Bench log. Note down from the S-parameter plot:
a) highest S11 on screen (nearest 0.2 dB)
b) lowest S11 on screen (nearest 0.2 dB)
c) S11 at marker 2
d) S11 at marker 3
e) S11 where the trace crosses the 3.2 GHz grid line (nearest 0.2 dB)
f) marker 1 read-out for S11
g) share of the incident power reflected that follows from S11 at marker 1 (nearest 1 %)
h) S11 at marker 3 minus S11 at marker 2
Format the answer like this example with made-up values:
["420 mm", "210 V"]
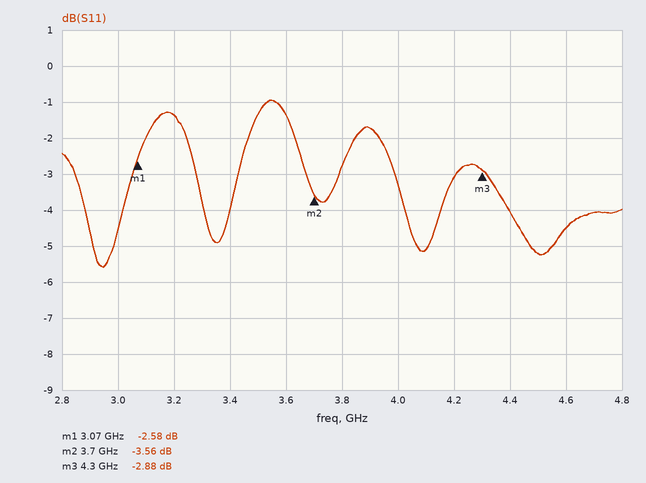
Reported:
["-1.0 dB", "-5.6 dB", "-3.56 dB", "-2.88 dB", "-1.4 dB", "-2.58 dB", "55 %", "0.68 dB"]
